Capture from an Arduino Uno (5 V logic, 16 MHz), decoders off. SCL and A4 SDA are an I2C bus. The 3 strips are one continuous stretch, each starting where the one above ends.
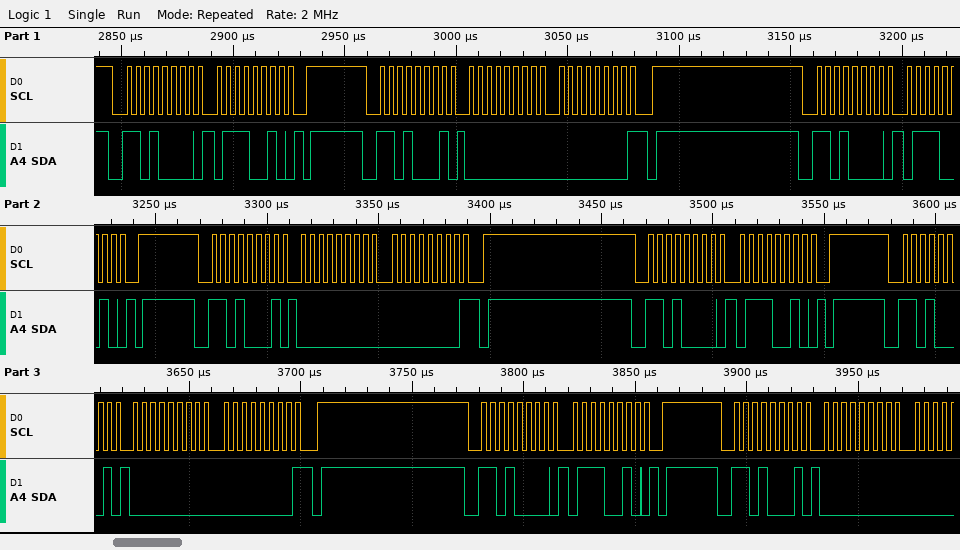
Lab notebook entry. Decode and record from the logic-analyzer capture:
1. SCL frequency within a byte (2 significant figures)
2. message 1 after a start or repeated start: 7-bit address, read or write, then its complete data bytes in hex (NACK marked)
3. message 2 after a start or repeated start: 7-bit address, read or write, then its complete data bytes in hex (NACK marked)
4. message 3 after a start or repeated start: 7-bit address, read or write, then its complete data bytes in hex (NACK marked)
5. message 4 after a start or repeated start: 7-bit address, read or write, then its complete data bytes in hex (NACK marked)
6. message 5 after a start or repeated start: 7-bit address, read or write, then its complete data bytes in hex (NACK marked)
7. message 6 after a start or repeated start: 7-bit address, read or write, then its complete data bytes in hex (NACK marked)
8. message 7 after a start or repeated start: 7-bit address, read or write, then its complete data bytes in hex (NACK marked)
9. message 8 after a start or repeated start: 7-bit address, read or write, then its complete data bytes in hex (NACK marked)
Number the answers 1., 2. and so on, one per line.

1. 250 kHz
2. 0x68 write: 72
3. 0x68 read: 00 00 NACK
4. 0x68 write: 72
5. 0x68 read: 00 00 NACK
6. 0x68 write: 72
7. 0x68 read: 00 00 NACK
8. 0x68 write: 72
9. 0x68 read: 00
